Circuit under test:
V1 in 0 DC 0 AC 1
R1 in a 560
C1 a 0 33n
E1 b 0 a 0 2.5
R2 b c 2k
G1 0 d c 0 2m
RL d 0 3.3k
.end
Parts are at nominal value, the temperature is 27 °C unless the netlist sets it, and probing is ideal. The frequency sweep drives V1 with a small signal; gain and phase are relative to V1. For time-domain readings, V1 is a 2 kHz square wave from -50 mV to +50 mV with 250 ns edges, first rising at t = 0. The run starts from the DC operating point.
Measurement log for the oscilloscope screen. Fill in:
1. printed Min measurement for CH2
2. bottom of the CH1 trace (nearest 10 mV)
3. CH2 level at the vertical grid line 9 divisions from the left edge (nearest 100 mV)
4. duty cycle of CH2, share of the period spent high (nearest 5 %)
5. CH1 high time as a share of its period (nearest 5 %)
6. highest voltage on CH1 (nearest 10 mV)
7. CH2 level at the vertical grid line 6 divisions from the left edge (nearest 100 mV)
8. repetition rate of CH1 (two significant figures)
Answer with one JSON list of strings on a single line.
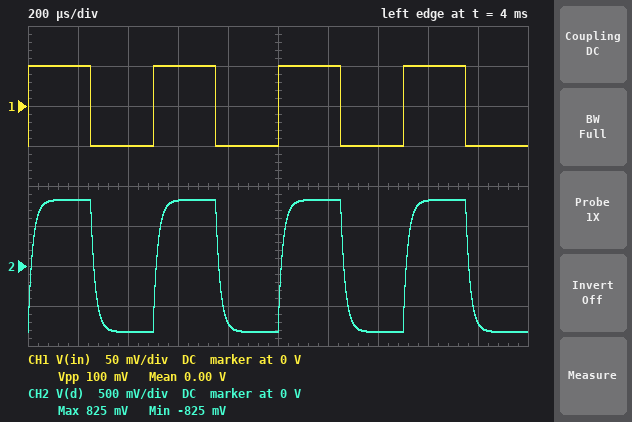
["-825 mV", "-50 mV", "-700 mV", "50 %", "50 %", "50 mV", "800 mV", "2.0 kHz"]
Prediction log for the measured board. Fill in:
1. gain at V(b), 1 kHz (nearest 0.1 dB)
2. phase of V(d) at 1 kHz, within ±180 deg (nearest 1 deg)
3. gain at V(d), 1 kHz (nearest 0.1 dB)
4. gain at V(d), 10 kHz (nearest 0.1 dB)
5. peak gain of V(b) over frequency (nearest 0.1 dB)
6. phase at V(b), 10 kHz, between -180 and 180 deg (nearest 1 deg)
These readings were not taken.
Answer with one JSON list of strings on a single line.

["7.9 dB", "-7 deg", "24.3 dB", "20.6 dB", "8.0 dB", "-49 deg"]
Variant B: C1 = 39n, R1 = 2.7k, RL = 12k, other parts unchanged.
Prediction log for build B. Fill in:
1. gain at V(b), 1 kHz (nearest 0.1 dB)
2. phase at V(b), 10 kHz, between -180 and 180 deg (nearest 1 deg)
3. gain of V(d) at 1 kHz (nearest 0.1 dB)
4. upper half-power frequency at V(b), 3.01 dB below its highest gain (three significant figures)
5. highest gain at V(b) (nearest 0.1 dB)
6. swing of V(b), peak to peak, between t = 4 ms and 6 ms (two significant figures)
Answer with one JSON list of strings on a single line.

["6.4 dB", "-81 deg", "34.0 dB", "1.51 kHz", "8.0 dB", "210 mV"]
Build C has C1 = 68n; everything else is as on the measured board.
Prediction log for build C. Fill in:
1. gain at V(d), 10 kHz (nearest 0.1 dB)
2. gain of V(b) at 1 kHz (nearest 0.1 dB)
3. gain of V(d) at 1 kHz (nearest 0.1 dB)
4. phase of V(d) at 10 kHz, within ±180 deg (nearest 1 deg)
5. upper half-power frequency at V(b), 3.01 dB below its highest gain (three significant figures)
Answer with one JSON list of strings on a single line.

["16.1 dB", "7.7 dB", "24.1 dB", "-67 deg", "4.18 kHz"]
